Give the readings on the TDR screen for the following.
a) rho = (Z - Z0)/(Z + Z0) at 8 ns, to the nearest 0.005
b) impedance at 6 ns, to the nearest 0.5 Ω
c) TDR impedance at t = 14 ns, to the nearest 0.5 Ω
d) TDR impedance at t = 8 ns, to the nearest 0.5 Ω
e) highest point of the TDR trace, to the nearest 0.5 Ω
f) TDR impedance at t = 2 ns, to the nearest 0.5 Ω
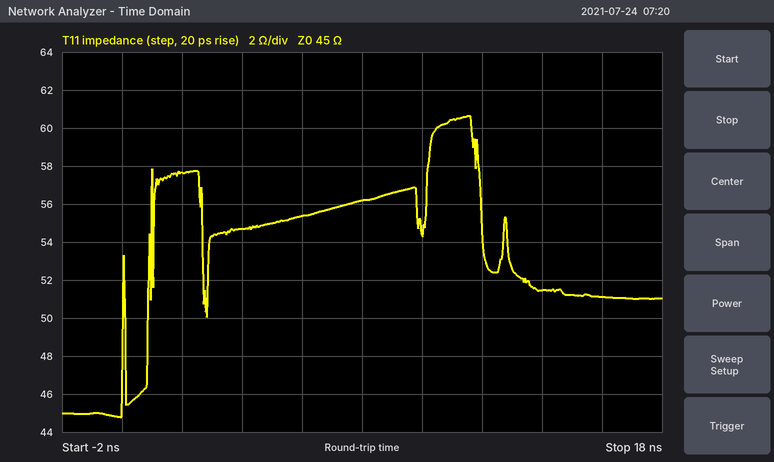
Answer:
+0.110
55.5 Ω
51.5 Ω
56.0 Ω
60.5 Ω
57.5 Ω
